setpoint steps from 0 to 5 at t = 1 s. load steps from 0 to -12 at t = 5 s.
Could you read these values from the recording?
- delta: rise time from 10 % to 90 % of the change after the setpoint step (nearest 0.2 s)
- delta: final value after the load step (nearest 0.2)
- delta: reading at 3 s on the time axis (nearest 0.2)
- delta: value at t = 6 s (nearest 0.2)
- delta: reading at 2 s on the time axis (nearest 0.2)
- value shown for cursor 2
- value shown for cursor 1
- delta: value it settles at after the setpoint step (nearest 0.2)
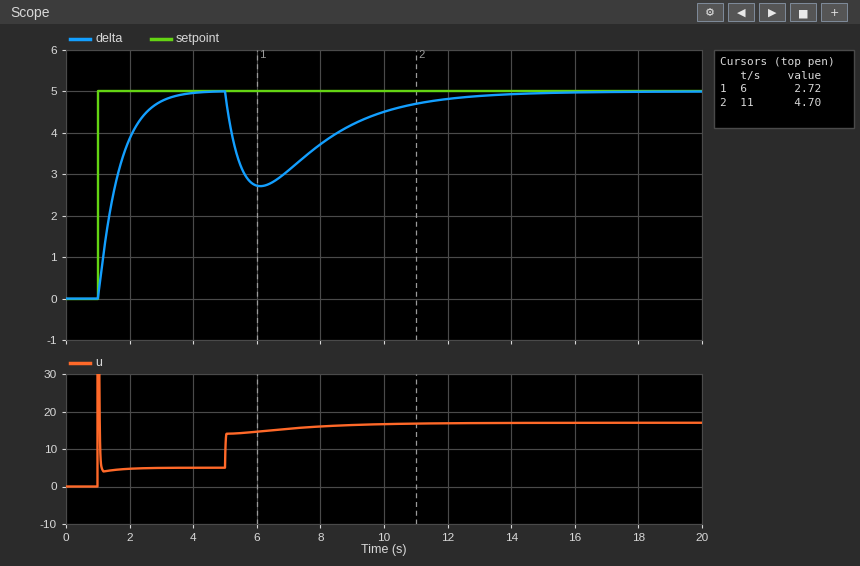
1.4 s
5.0
4.8
2.8
3.8
4.70
2.72
5.0
